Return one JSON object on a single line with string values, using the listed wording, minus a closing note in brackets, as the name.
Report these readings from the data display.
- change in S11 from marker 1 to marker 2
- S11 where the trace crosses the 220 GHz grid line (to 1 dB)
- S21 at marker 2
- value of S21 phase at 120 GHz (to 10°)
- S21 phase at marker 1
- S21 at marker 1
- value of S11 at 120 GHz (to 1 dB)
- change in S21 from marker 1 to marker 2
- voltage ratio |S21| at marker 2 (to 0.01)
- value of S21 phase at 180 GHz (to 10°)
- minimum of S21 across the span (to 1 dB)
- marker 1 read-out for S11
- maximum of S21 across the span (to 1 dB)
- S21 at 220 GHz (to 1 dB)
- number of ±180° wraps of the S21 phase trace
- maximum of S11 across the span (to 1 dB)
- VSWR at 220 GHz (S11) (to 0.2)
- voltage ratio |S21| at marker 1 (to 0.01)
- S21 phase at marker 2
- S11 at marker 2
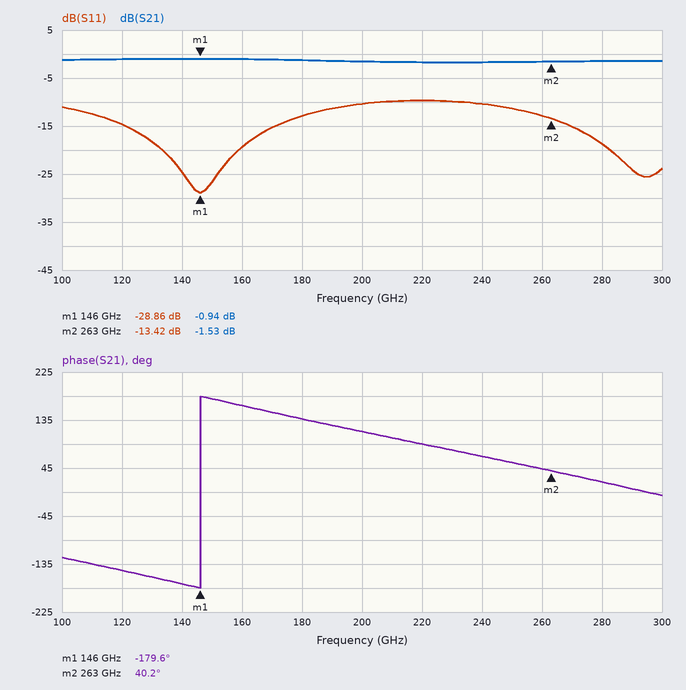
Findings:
{"change in S11 from marker 1 to marker 2": "15.44 dB", "S11 where the trace crosses the 220 GHz grid line": "-10 dB", "S21 at marker 2": "-1.53 dB", "value of S21 phase at 120 GHz": "-150°", "S21 phase at marker 1": "-179.6°", "S21 at marker 1": "-0.94 dB", "value of S11 at 120 GHz": "-15 dB", "change in S21 from marker 1 to marker 2": "-0.59 dB", "voltage ratio |S21| at marker 2": "0.84", "value of S21 phase at 180 GHz": "140°", "minimum of S21 across the span": "-2 dB", "marker 1 read-out for S11": "-28.86 dB", "maximum of S21 across the span": "-1 dB", "S21 at 220 GHz": "-2 dB", "number of ±180° wraps of the S21 phase trace": "1", "maximum of S11 across the span": "-10 dB", "VSWR at 220 GHz (S11)": "2.0", "voltage ratio |S21| at marker 1": "0.90", "S21 phase at marker 2": "40.2°", "S11 at marker 2": "-13.42 dB"}
